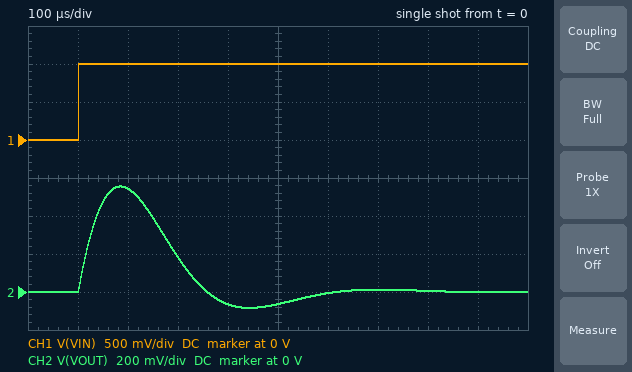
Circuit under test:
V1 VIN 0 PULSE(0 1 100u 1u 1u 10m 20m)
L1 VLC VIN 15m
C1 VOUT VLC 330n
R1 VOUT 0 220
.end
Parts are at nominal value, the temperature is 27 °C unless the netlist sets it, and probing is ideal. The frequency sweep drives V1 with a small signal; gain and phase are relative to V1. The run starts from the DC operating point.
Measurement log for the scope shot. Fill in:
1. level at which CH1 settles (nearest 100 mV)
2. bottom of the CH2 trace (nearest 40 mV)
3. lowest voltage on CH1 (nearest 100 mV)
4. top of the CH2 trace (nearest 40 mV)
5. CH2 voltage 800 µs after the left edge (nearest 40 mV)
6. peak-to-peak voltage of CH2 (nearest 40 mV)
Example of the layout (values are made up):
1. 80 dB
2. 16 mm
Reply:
1. 1.0 V
2. -80 mV
3. 0 V
4. 560 mV
5. 0 V
6. 640 mV
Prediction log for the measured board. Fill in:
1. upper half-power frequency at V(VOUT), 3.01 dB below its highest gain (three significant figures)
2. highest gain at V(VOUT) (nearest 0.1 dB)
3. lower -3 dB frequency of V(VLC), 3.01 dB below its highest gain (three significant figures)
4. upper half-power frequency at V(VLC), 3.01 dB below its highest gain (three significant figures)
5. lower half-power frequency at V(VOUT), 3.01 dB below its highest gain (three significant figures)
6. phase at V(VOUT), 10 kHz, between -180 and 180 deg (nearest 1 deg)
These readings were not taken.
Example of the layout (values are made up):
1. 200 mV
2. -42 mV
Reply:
1. 3.71 kHz
2. 0 dB
3. 339 Hz
4. 3.14 kHz
5. 1.38 kHz
6. -76 deg
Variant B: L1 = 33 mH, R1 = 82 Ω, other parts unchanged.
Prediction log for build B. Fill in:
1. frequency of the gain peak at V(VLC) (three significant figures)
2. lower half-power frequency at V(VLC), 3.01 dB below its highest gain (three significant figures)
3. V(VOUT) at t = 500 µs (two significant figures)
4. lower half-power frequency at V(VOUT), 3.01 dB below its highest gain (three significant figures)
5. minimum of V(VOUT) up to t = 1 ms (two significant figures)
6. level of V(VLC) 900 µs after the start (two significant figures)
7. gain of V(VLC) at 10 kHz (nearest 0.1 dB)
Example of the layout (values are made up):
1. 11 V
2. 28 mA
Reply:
1. 1.50 kHz
2. 1.29 kHz
3. -97 mV
4. 1.34 kHz
5. -140 mV
6. 950 mV
7. -26.6 dB
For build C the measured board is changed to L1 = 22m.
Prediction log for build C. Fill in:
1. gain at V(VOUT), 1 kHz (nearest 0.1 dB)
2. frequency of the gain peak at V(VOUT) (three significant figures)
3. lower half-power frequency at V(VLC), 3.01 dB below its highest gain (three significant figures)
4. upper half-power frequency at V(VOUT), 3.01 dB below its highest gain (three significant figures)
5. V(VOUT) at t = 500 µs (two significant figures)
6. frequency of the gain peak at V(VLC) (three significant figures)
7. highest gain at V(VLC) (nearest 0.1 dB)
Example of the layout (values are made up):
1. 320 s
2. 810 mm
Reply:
1. -5.4 dB
2. 1.87 kHz
3. 661 Hz
4. 2.83 kHz
5. -110 mV
6. 1.65 kHz
7. 4.1 dB
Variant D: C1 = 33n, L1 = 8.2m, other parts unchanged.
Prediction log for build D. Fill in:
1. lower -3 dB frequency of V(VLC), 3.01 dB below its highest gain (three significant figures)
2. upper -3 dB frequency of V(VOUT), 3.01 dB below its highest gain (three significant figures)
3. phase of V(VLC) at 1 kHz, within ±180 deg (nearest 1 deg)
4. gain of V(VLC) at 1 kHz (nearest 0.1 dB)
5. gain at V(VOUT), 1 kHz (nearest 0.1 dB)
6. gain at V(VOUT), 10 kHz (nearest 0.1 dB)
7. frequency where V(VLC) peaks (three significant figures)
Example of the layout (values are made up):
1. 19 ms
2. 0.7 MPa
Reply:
1. 6.86 kHz
2. 12.0 kHz
3. 0 deg
4. 0.1 dB
5. -26.7 dB
6. -0.1 dB
7. 9.27 kHz
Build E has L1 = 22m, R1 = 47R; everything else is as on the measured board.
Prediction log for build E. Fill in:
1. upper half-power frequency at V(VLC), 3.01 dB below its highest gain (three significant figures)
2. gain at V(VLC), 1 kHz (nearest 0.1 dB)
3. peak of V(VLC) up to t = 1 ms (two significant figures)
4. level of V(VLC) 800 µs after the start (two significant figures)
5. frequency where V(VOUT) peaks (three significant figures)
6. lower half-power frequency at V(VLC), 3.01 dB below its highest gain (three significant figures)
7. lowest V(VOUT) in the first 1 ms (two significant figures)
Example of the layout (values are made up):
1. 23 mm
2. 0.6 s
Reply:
1. 2.02 kHz
2. 2.9 dB
3. 1.8 V
4. 1.2 V
5. 1.87 kHz
6. 1.67 kHz
7. -120 mV
